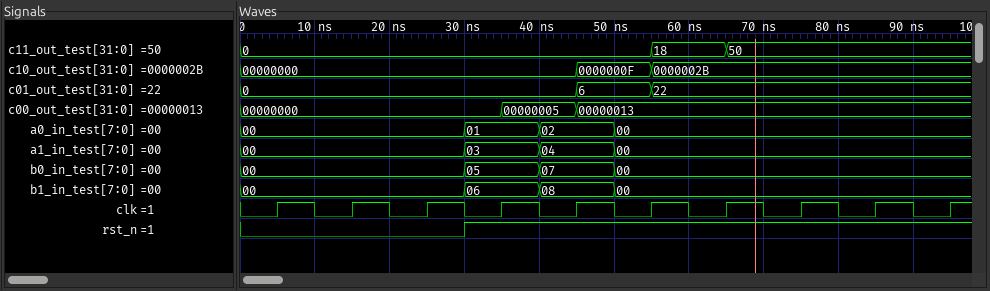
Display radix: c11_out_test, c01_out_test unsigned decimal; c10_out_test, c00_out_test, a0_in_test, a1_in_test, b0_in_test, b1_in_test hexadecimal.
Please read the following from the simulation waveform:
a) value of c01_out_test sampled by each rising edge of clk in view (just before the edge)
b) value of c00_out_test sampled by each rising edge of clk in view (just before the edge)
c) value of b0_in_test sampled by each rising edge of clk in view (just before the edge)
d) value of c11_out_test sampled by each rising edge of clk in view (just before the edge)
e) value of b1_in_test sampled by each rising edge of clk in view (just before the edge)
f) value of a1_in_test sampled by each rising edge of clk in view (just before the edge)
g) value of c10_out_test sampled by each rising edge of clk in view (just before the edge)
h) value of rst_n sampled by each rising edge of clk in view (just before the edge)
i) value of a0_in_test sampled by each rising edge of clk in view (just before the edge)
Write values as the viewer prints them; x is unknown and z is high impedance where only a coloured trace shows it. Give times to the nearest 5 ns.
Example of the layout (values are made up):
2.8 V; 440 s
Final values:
0, 0, 0, 0, 0, 6, 22, 22, 22, 22; 00000000, 00000000, 00000000, 00000000, 00000005, 00000013, 00000013, 00000013, 00000013, 00000013; 00, 00, 00, 05, 07, 00, 00, 00, 00, 00; 0, 0, 0, 0, 0, 0, 18, 50, 50, 50; 00, 00, 00, 06, 08, 00, 00, 00, 00, 00; 00, 00, 00, 03, 04, 00, 00, 00, 00, 00; 00000000, 00000000, 00000000, 00000000, 00000000, 0000000F, 0000002B, 0000002B, 0000002B, 0000002B; 0 0 0 1 1 1 1 1 1 1; 00, 00, 00, 01, 02, 00, 00, 00, 00, 00
